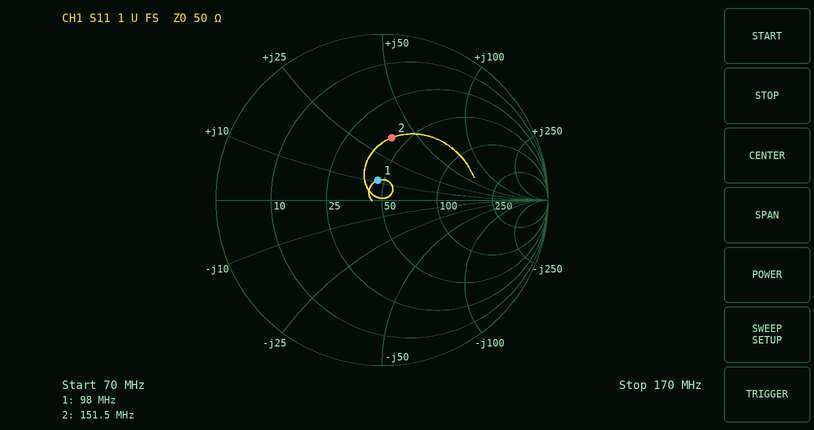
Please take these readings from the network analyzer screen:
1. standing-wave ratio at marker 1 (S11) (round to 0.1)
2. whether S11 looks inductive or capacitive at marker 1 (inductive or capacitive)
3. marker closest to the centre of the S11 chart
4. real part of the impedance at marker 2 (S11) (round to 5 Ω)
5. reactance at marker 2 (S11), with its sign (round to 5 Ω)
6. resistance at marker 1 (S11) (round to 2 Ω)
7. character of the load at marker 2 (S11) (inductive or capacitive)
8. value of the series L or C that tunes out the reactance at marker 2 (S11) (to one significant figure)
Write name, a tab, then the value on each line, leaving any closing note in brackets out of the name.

standing-wave ratio at marker 1 (S11)	1.3
whether S11 looks inductive or capacitive at marker 1	inductive
marker closest to the centre of the S11 chart	marker 1
real part of the impedance at marker 2 (S11)	40 Ω
reactance at marker 2 (S11), with its sign	+35 Ω
resistance at marker 1 (S11)	46 Ω
character of the load at marker 2 (S11)	inductive
value of the series L or C that tunes out the reactance at marker 2 (S11)	30 pF
